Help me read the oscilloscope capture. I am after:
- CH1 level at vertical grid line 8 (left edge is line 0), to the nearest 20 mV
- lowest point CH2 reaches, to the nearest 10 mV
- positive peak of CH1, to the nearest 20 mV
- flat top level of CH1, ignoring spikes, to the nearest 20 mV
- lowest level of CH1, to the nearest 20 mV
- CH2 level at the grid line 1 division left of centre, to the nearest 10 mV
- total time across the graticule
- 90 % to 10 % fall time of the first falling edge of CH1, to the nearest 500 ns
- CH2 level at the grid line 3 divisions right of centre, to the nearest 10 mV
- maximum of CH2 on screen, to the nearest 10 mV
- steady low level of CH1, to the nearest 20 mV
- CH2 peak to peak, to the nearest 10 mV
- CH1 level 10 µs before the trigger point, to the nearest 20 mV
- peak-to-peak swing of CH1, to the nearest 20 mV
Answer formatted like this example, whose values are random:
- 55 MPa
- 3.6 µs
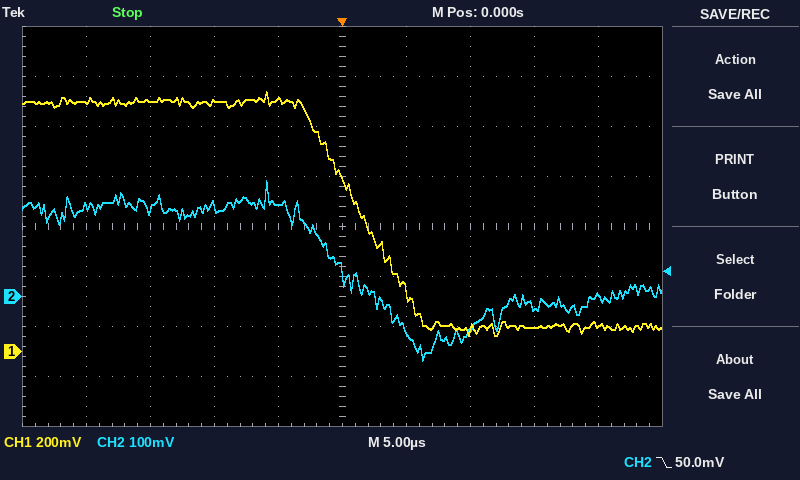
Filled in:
- 100 mV
- -130 mV
- 1.04 V
- 1.00 V
- 60 mV
- 180 mV
- 50 µs
- 8.0 µs
- -20 mV
- 230 mV
- 100 mV
- 360 mV
- 1.00 V
- 980 mV
